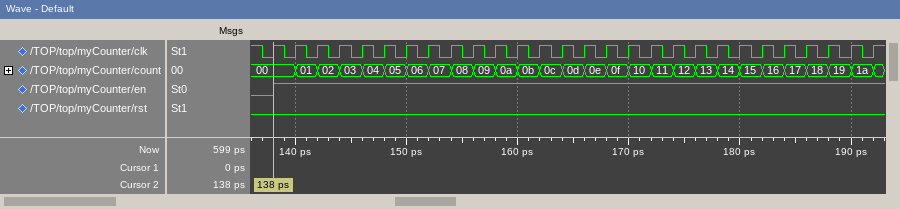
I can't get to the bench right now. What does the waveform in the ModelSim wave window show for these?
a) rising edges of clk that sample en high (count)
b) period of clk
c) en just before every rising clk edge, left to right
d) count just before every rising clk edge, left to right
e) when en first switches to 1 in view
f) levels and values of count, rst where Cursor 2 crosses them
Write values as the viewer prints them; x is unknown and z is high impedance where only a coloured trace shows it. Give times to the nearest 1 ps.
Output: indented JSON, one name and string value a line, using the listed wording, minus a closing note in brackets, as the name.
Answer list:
{
  "rising edges of clk that sample en high": "27",
  "period of clk": "2 ps",
  "en just before every rising clk edge, left to right": "0 1 1 1 1 1 1 1 1 1 1 1 1 1 1 1 1 1 1 1 1 1 1 1 1 1 1 1",
  "count just before every rising clk edge, left to right": "00, 00, 01, 02, 03, 04, 05, 06, 07, 08, 09, 0a, 0b, 0c, 0d, 0e, 0f, 10, 11, 12, 13, 14, 15, 16, 17, 18, 19, 1a",
  "when en first switches to 1 in view": "138 ps",
  "levels and values of count, rst where Cursor 2 crosses them": "count=00, rst=0"
}
